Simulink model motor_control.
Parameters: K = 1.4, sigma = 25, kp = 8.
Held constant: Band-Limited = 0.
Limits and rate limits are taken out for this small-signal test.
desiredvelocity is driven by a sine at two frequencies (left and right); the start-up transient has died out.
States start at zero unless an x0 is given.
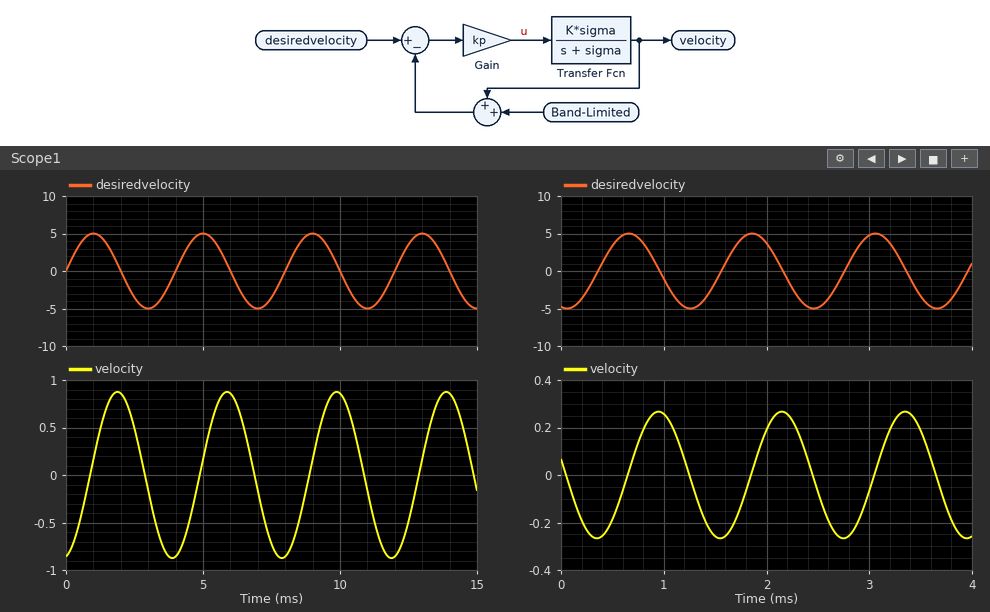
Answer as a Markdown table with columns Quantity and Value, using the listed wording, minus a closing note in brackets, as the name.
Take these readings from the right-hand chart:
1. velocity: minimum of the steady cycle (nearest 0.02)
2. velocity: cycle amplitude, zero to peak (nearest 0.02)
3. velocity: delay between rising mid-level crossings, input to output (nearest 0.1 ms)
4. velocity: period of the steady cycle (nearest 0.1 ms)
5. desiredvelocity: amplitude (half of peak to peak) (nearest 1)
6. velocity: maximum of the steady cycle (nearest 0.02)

| Quantity | Value |
|---|---|
| velocity: minimum of the steady cycle | -0.26 |
| velocity: cycle amplitude, zero to peak | 0.26 |
| velocity: delay between rising mid-level crossings, input to output | 0.3 ms |
| velocity: period of the steady cycle | 1.2 ms |
| desiredvelocity: amplitude (half of peak to peak) | 5 |
| velocity: maximum of the steady cycle | 0.26 |
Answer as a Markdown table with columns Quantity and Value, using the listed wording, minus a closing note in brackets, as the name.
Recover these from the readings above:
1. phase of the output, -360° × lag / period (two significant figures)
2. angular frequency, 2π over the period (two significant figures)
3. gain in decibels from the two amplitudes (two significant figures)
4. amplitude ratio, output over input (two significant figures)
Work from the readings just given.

| Quantity | Value |
|---|---|
| phase of the output, -360° × lag / period | -90° |
| angular frequency, 2π over the period | 5.2 rad/ms |
| gain in decibels from the two amplitudes | -26 dB |
| amplitude ratio, output over input | 0.052 |
